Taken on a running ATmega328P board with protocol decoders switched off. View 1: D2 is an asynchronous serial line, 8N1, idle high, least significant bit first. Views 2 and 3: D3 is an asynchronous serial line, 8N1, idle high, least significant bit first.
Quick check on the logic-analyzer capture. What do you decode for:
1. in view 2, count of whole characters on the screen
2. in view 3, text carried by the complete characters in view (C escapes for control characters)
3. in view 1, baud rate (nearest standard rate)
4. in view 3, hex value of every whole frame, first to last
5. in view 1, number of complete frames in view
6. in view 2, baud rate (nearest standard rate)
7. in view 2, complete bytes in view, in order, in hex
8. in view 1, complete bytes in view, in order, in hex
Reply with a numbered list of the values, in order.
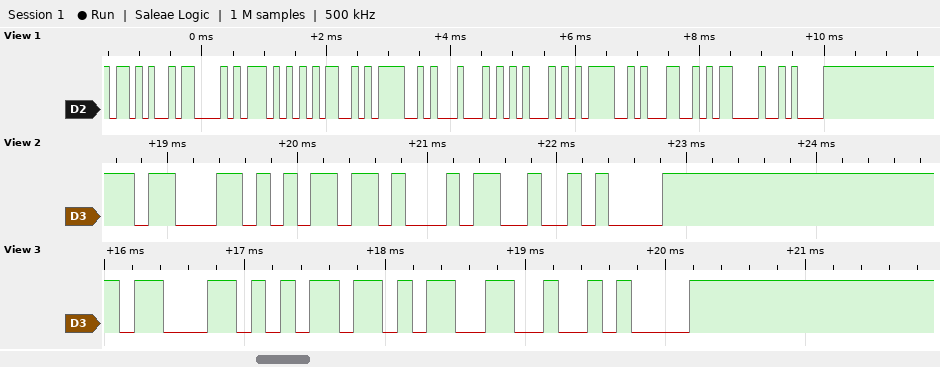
1. 4
2. "cm3\n"
3. 9600 baud
4. 63 6D 33 0A
5. 11
6. 9600 baud
7. 63 6D 34 0A
8. 2B 43 57 4D 4F 44 45 3D 31 0D 0A
